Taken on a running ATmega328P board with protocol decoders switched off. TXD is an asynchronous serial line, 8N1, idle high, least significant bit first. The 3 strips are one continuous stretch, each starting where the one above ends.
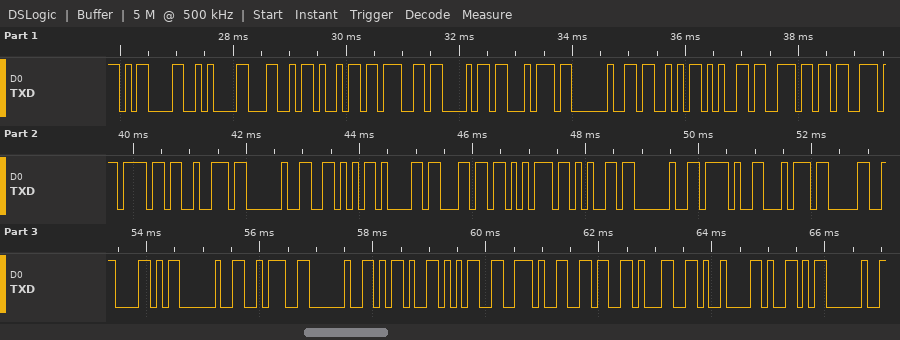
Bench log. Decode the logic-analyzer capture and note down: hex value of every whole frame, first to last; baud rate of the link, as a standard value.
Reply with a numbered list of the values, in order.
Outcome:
1. 0D 0A 4C 69 67 68 74 20 53 65 6E 73 6F 72 20 56 61 6C 75 65 20 2F 74 30 58 20 3A 20 2D 35 2E 36 31 09 59 20
2. 9600 baud
